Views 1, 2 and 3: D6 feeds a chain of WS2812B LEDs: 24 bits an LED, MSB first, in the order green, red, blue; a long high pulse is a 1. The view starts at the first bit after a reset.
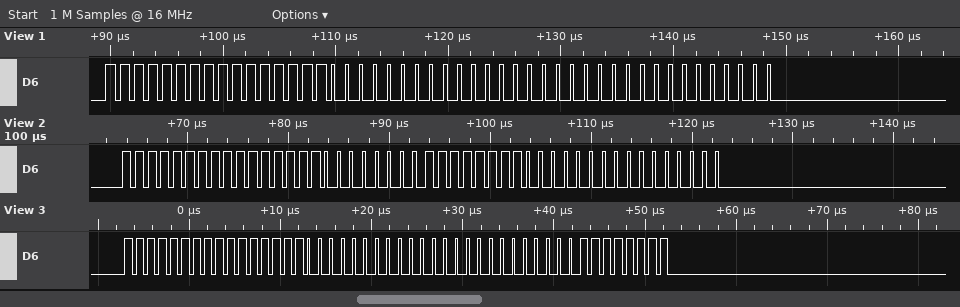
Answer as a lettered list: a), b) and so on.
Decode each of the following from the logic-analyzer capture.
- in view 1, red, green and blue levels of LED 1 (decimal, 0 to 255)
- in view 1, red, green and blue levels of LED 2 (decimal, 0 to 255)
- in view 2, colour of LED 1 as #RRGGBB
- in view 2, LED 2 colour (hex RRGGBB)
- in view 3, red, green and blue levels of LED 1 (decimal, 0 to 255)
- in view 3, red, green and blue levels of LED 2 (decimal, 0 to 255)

a) 255, 255, 0
b) 0, 0, 0
c) #FFFF00
d) #00FF00
e) 255, 255, 0
f) 0, 0, 255
